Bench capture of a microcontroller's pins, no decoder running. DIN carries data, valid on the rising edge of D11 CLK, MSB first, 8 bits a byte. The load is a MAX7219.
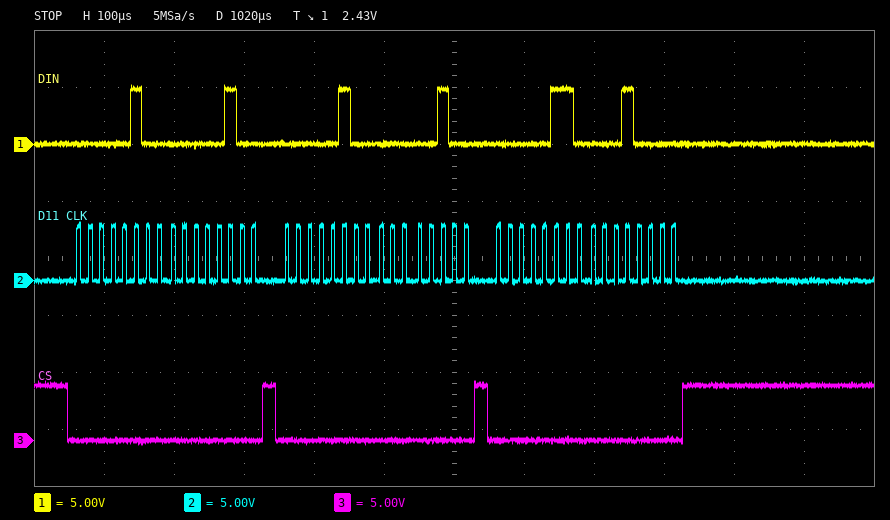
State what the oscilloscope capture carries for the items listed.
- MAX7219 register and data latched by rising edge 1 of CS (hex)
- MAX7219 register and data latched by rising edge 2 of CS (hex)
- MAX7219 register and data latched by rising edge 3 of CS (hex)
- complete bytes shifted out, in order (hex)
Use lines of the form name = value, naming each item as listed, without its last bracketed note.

MAX7219 register and data latched by rising edge 1 of CS = register 0x4, data 0x04
MAX7219 register and data latched by rising edge 2 of CS = register 0x4, data 0x04
MAX7219 register and data latched by rising edge 3 of CS = register 0x6, data 0x10
complete bytes shifted out, in order = 0x04 0x04 0x04 0x04 0x06 0x10
